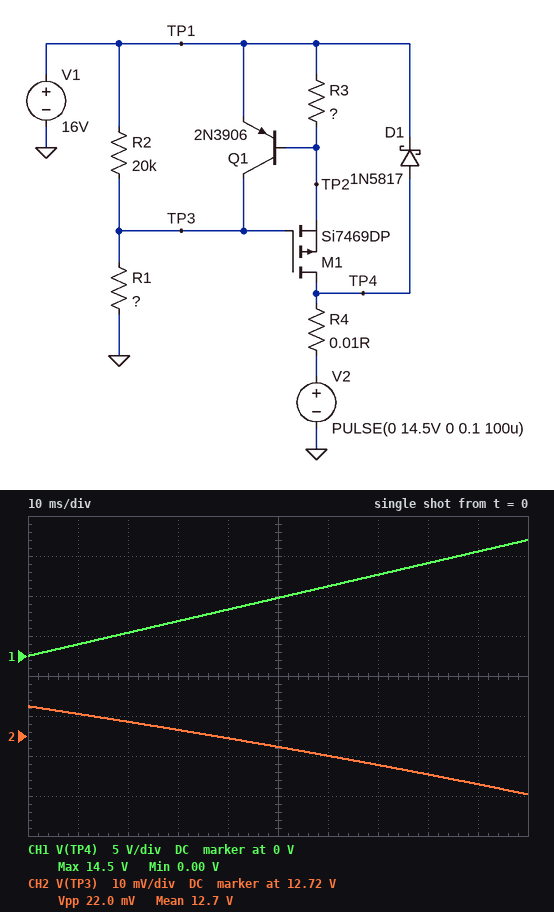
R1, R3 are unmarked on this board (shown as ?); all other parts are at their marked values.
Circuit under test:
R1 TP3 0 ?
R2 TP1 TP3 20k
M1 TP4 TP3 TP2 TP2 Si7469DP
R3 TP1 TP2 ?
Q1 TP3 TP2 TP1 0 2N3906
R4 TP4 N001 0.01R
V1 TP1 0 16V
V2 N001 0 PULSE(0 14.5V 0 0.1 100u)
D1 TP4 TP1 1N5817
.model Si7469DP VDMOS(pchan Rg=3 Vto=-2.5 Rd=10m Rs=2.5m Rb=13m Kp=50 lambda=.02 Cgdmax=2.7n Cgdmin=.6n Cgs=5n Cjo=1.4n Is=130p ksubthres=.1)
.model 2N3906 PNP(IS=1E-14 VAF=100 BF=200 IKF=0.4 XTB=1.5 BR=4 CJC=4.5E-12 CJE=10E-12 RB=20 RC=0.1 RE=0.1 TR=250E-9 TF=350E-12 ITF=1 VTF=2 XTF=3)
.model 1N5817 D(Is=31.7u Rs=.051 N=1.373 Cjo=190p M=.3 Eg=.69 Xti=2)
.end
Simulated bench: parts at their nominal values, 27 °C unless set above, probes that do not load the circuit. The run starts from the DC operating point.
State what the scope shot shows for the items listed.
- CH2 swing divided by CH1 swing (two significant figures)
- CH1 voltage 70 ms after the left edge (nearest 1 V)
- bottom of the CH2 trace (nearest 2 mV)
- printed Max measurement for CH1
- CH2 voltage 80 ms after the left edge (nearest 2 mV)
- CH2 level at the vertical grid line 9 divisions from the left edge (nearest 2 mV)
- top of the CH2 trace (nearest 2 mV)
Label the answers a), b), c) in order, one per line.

a) 0.0015
b) 10 V
c) 12.706 V
d) 14.5 V
e) 12.710 V
f) 12.708 V
g) 12.728 V
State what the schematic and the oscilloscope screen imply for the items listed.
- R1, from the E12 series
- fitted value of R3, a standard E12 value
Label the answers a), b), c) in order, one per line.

a) 3.3 kΩ
b) 1.5 Ω
